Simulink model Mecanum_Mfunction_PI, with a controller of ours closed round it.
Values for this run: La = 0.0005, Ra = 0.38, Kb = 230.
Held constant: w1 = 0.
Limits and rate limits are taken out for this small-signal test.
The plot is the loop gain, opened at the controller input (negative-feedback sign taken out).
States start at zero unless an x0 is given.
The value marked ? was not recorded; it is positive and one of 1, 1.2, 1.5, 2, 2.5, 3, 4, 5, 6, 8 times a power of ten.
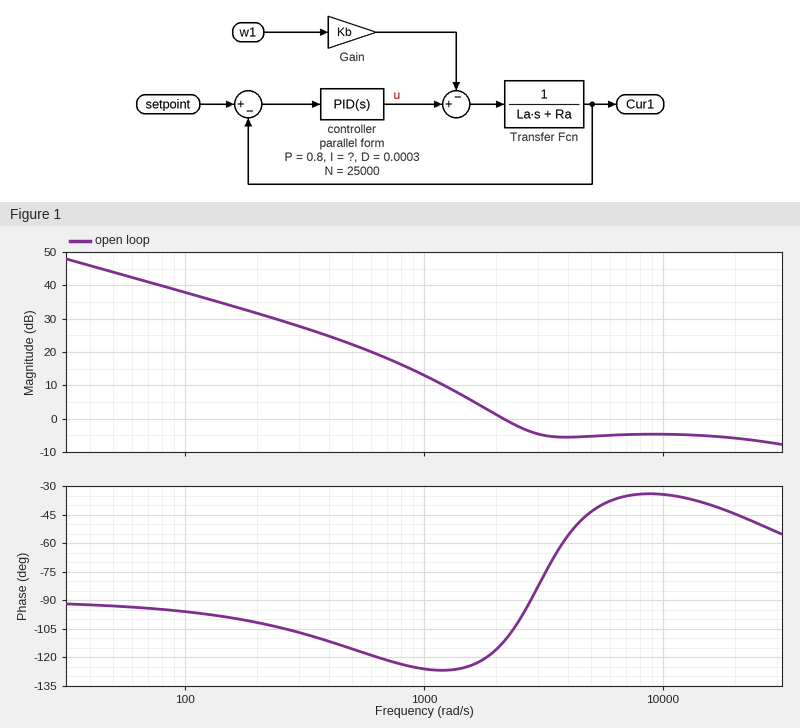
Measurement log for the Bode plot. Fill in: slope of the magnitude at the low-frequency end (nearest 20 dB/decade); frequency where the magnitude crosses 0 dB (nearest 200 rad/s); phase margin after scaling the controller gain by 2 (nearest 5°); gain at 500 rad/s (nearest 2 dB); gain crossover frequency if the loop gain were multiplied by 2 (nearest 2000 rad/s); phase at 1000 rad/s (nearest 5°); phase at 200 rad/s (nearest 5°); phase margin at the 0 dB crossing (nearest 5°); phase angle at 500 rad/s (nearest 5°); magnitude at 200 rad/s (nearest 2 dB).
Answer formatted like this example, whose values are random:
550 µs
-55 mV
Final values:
-20 dB/decade
2200 rad/s
135°
22 dB
22000 rad/s
-125°
-100°
70°
-115°
32 dB
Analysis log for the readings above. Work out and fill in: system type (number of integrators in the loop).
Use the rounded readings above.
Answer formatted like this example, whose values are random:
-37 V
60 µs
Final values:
1
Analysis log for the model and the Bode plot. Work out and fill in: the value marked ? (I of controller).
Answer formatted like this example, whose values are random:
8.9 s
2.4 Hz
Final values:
3000
